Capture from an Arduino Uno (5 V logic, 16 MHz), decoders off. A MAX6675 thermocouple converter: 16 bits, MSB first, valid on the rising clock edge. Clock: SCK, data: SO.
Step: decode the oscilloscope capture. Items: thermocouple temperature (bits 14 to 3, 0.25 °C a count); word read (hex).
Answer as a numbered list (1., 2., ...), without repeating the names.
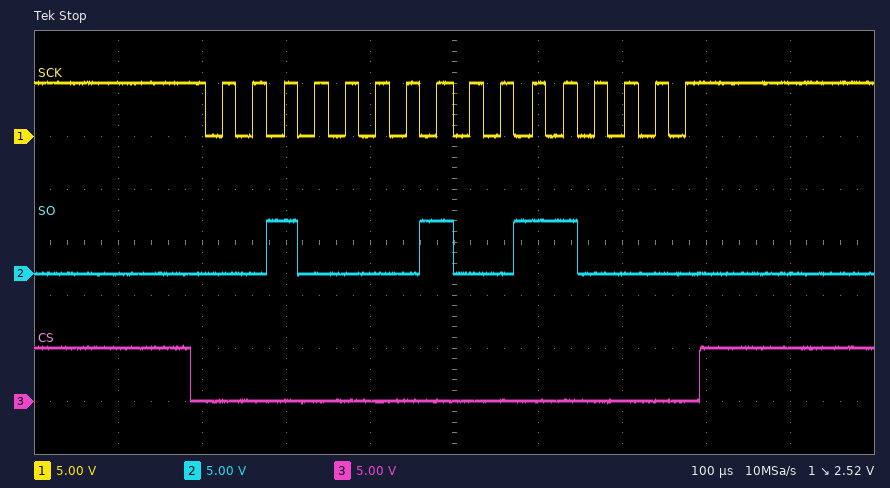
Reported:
1. 265.50 °C
2. 0x2130
